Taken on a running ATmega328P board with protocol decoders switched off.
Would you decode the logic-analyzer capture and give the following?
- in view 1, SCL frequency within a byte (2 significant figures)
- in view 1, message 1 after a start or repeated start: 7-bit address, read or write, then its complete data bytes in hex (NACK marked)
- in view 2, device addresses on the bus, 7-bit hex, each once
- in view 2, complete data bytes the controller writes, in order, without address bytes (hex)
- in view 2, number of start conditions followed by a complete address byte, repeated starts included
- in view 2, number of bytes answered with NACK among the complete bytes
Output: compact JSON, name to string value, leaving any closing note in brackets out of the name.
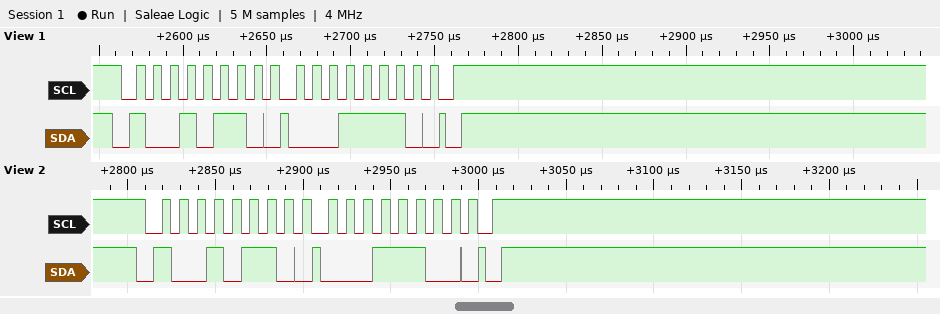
{"in view 1, SCL frequency within a byte": "100 kHz", "in view 1, message 1 after a start or repeated start: 7-bit address, read or write, then its complete data bytes in hex": "0x4B write: 1E", "in view 2, device addresses on the bus, 7-bit hex, each once": "0x4B", "in view 2, complete data bytes the controller writes, in order, without address bytes": "1C", "in view 2, number of start conditions followed by a complete address byte, repeated starts included": "1", "in view 2, number of bytes answered with NACK among the complete bytes": "0"}
